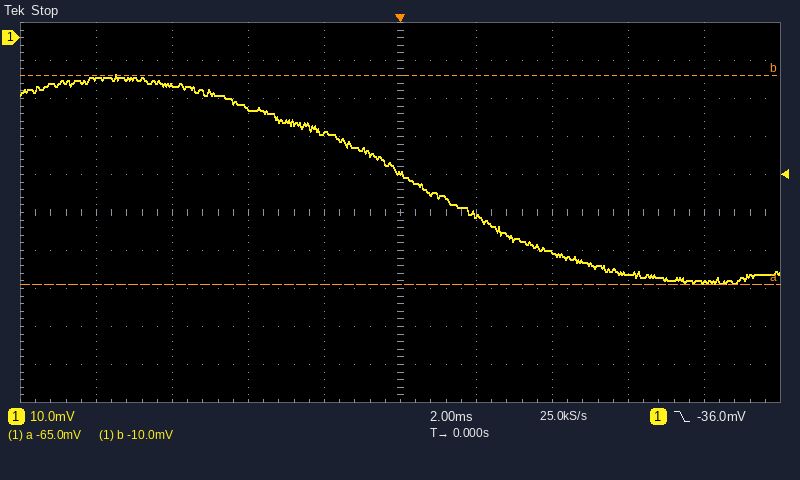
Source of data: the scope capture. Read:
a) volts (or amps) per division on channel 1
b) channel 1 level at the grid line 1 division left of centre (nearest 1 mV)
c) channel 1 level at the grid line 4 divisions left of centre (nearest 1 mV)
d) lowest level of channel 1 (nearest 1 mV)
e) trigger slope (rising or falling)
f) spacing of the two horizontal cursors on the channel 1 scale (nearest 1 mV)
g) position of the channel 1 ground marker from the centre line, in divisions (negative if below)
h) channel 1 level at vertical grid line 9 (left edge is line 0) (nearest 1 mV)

10 mV
-25 mV
-11 mV
-65 mV
falling
55 mV
+4.6 div
-64 mV
